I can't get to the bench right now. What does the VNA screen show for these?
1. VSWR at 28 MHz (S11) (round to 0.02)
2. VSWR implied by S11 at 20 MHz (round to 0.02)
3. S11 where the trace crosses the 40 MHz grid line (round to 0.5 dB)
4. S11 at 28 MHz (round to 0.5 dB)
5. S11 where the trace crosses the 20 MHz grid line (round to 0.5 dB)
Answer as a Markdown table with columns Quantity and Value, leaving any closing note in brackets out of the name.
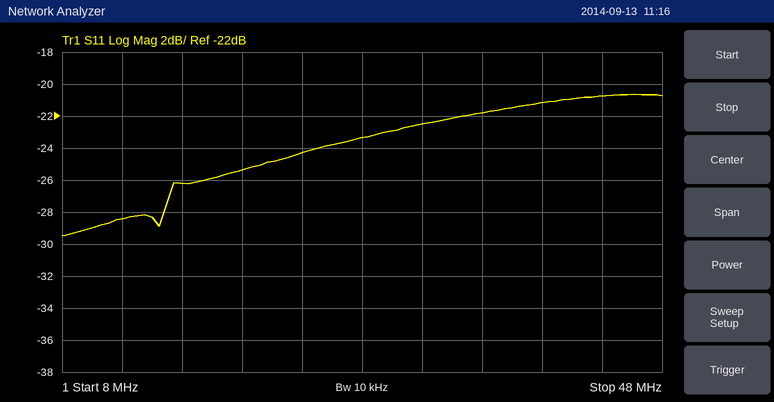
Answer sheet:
| Quantity | Value |
|---|---|
| VSWR at 28 MHz (S11) | 1.14 |
| VSWR implied by S11 at 20 MHz | 1.12 |
| S11 where the trace crosses the 40 MHz grid line | -21.0 dB |
| S11 at 28 MHz | -23.5 dB |
| S11 where the trace crosses the 20 MHz grid line | -25.5 dB |
